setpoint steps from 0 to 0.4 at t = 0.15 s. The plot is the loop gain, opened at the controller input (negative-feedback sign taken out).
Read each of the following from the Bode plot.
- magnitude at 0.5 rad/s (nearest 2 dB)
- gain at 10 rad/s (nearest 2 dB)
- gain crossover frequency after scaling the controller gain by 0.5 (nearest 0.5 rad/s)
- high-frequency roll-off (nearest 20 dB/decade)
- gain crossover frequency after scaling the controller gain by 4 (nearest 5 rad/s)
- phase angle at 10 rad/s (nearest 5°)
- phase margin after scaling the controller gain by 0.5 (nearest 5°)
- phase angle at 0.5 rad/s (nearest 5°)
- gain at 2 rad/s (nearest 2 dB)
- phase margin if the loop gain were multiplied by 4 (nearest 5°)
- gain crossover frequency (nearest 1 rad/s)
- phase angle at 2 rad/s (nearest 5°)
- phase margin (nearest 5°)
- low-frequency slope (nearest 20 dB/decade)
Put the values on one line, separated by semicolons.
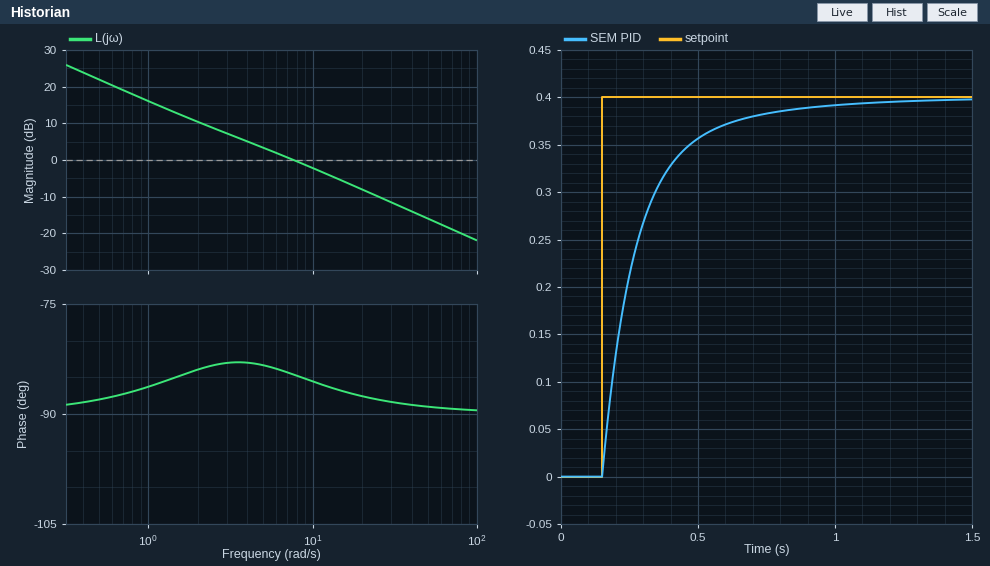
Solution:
22 dB; -2 dB; 3.5 rad/s; -20 dB/decade; 30 rad/s; -85°; 95°; -90°; 10 dB; 90°; 8 rad/s; -85°; 95°; -20 dB/decade
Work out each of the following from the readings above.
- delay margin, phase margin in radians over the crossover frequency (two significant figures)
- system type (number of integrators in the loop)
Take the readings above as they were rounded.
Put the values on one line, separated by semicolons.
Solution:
0.21 s; 1
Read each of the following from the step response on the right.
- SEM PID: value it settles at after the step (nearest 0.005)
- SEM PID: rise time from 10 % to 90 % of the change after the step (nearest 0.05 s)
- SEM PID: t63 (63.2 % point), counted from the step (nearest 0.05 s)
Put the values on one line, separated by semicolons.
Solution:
0.400; 0.35 s; 0.15 s
